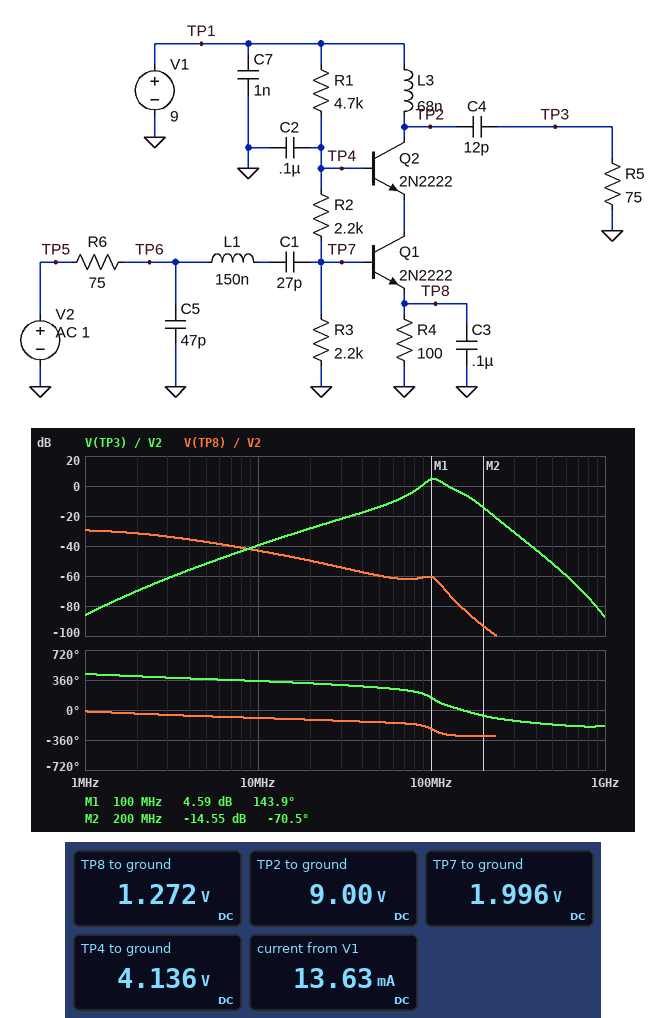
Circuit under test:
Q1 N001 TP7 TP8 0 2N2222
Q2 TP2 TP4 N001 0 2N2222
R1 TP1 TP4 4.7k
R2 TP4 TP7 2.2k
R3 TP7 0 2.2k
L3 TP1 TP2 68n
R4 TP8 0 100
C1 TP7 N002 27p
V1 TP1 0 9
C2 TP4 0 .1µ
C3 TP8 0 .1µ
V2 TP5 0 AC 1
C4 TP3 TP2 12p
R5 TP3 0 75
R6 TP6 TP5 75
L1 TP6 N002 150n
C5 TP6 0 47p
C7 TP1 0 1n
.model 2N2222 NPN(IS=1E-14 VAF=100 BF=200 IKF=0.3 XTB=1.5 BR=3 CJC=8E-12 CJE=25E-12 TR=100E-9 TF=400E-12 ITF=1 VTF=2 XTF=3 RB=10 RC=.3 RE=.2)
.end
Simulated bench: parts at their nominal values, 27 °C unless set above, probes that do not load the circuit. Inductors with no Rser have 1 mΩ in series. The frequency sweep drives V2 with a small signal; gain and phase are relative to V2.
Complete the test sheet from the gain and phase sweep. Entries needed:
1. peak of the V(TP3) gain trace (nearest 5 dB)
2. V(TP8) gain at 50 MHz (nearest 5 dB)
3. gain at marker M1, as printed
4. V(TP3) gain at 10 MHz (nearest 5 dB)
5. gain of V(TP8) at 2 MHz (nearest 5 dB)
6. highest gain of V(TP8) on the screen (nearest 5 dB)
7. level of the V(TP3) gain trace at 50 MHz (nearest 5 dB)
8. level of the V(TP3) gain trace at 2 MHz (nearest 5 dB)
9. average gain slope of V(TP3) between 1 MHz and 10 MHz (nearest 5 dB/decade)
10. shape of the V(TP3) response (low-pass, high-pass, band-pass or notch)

5 dB
-60 dB
4.59 dB
-40 dB
-30 dB
-30 dB
-15 dB
-70 dB
45 dB/decade
band-pass
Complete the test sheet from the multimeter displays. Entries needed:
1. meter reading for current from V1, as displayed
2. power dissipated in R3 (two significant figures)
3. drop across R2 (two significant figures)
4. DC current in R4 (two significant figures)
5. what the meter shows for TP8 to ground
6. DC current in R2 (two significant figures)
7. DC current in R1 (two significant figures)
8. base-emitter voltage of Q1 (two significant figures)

13.63 mA
1.8 mW
2.1 V
13 mA
1.272 V
970 µA
1.0 mA
720 mV
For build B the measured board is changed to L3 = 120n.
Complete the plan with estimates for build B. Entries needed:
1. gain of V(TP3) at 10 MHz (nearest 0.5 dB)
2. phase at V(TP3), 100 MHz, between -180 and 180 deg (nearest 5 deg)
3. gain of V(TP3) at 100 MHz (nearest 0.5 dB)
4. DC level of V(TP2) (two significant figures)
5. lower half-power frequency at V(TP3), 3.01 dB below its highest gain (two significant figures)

-34.5 dB
120 deg
13.0 dB
9.0 V
92 MHz
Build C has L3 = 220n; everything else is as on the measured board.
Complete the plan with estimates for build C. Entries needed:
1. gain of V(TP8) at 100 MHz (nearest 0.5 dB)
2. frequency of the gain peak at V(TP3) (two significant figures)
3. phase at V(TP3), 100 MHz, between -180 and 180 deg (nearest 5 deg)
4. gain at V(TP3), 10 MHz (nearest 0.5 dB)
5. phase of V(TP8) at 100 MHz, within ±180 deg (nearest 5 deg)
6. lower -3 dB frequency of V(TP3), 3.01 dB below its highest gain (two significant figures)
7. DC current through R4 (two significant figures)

-61.0 dB
94 MHz
45 deg
-29.5 dB
125 deg
81 MHz
13 mA
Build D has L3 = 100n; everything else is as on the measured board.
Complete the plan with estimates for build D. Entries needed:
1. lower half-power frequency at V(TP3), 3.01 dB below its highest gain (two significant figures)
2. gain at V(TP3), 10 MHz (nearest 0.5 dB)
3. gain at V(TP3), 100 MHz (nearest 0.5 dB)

92 MHz
-36.0 dB
10.0 dB
